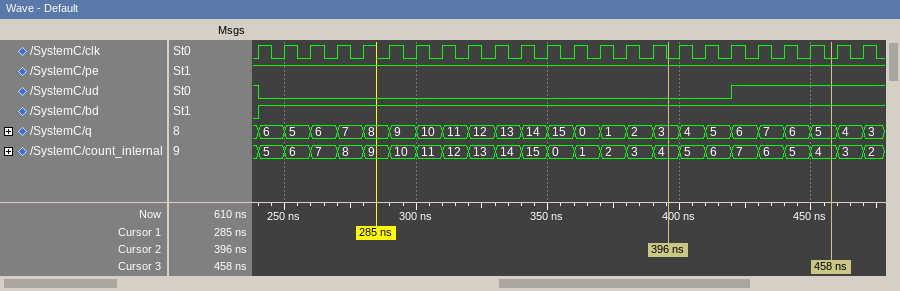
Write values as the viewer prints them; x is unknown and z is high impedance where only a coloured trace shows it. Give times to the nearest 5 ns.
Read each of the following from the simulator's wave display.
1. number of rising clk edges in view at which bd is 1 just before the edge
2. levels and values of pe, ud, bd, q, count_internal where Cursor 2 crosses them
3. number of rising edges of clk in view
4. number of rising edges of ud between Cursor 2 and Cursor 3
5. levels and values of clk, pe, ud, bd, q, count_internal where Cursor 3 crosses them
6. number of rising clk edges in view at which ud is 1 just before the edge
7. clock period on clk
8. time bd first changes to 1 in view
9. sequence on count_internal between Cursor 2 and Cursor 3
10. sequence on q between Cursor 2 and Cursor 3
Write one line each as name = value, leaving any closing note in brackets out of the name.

number of rising clk edges in view at which bd is 1 just before the edge = 23
levels and values of pe, ud, bd, q, count_internal where Cursor 2 crosses them = pe=1, ud=0, bd=1, q=3, count_internal=4
number of rising edges of clk in view = 24
number of rising edges of ud between Cursor 2 and Cursor 3 = 1
levels and values of clk, pe, ud, bd, q, count_internal where Cursor 3 crosses them = clk=0, pe=1, ud=1, bd=1, q=5, count_internal=4
number of rising clk edges in view at which ud is 1 just before the edge = 6
clock period on clk = 10 ns
time bd first changes to 1 in view = 240 ns
sequence on count_internal between Cursor 2 and Cursor 3 = 4, 5, 6, 7, 6, 5, 4
sequence on q between Cursor 2 and Cursor 3 = 3, 4, 5, 6, 7, 6, 5
